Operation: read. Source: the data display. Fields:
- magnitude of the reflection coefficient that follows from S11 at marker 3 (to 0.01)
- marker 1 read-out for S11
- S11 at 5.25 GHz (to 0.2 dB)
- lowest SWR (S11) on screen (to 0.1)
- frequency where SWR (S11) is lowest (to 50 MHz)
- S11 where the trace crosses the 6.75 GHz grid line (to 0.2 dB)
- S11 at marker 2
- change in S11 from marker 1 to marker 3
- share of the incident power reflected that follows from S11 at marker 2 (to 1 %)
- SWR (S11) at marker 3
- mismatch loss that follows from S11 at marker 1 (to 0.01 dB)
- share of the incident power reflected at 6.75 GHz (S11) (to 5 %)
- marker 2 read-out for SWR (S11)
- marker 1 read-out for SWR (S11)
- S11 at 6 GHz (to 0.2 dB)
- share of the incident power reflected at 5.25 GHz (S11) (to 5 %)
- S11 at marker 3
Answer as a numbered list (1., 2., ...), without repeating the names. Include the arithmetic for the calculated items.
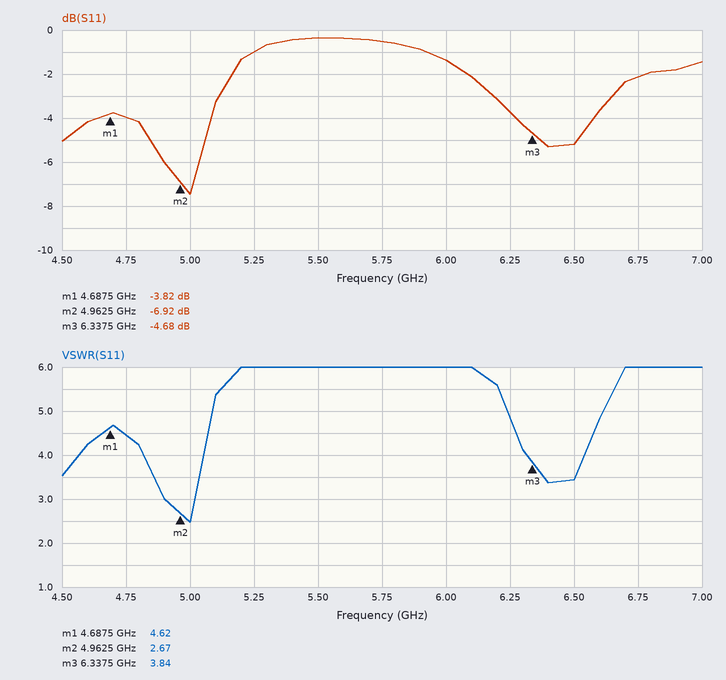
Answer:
1. 10^(-4.68/20) ≈ 0.58
2. -3.82 dB
3. -1.0 dB
4. 2.5
5. 5.00 GHz
6. -2.2 dB
7. -6.92 dB
8. -4.68 − (-3.82) = -0.86 dB
9. 10^(-6.92/10) ≈ 20 %
10. 3.84
11. −10 log10(1 − 10^(-3.82/10)) ≈ 2.33 dB
12. 10^(-2.2/10) ≈ 60 %
13. 2.67
14. 4.62
15. -1.4 dB
16. 10^(-1/10) ≈ 79.4 %, so 80 % to the nearest 5 %
17. -4.68 dB
